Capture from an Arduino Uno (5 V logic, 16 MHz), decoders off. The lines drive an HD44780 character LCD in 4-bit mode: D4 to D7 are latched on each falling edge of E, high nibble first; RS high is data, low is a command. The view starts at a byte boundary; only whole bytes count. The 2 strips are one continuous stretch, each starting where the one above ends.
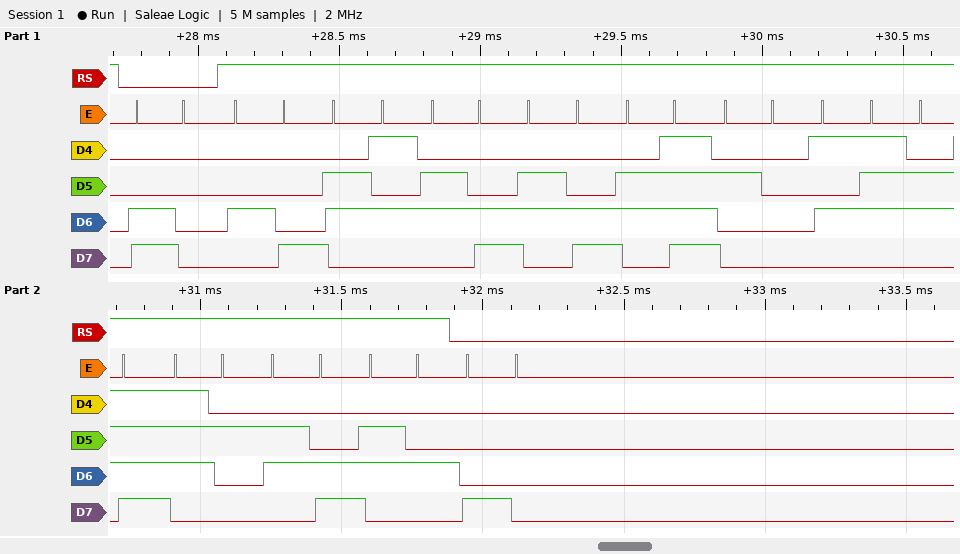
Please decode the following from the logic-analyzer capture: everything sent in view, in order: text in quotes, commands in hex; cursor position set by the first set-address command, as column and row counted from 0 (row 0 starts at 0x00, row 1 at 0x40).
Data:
0xC0 "Hello World" 0x80
column 0, row 1
